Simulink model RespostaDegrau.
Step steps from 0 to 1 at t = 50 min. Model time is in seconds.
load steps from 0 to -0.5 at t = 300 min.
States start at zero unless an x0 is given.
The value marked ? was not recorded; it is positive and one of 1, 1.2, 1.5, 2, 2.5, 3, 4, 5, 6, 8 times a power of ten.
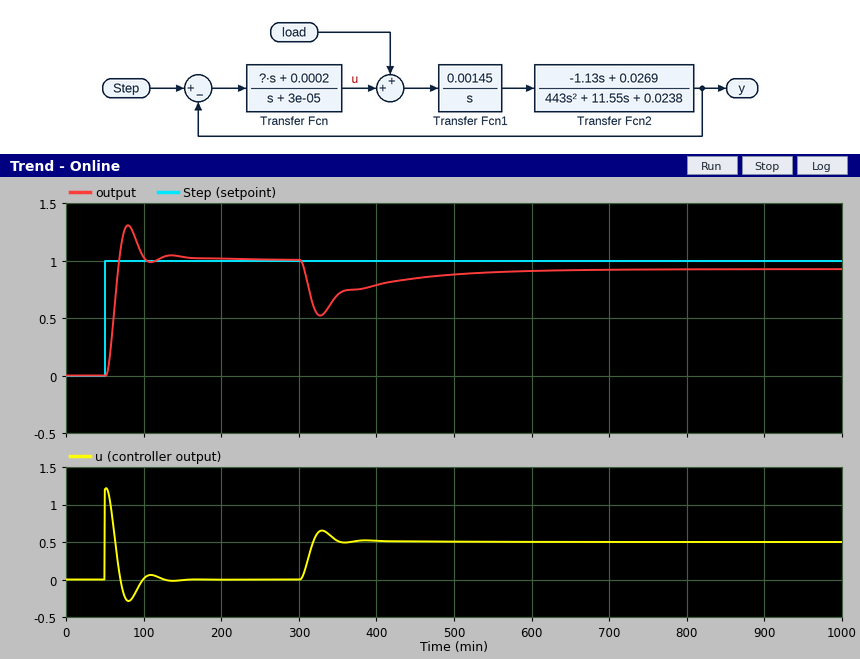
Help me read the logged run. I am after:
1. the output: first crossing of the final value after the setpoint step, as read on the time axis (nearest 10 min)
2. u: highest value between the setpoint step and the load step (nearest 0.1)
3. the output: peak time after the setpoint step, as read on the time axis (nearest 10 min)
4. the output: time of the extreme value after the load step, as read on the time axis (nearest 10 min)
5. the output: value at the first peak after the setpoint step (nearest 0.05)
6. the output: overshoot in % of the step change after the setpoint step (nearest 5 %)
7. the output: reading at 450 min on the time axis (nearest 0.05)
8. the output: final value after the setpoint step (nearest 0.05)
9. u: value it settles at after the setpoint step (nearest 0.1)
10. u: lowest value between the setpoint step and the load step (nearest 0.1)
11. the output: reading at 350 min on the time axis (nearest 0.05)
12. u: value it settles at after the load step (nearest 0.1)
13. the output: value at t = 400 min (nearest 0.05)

70 min
1.2
80 min
330 min
1.30
30 %
0.85
1.00
0.0
-0.3
0.70
0.5
0.80
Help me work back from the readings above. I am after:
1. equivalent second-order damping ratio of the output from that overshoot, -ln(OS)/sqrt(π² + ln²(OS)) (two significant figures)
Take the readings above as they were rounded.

0.36
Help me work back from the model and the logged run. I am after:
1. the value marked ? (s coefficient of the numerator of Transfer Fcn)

1.2
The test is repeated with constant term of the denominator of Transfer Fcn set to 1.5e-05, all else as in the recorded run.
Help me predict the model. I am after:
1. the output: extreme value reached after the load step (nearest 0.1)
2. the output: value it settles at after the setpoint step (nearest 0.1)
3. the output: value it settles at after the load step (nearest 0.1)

0.5
1.0
1.0
